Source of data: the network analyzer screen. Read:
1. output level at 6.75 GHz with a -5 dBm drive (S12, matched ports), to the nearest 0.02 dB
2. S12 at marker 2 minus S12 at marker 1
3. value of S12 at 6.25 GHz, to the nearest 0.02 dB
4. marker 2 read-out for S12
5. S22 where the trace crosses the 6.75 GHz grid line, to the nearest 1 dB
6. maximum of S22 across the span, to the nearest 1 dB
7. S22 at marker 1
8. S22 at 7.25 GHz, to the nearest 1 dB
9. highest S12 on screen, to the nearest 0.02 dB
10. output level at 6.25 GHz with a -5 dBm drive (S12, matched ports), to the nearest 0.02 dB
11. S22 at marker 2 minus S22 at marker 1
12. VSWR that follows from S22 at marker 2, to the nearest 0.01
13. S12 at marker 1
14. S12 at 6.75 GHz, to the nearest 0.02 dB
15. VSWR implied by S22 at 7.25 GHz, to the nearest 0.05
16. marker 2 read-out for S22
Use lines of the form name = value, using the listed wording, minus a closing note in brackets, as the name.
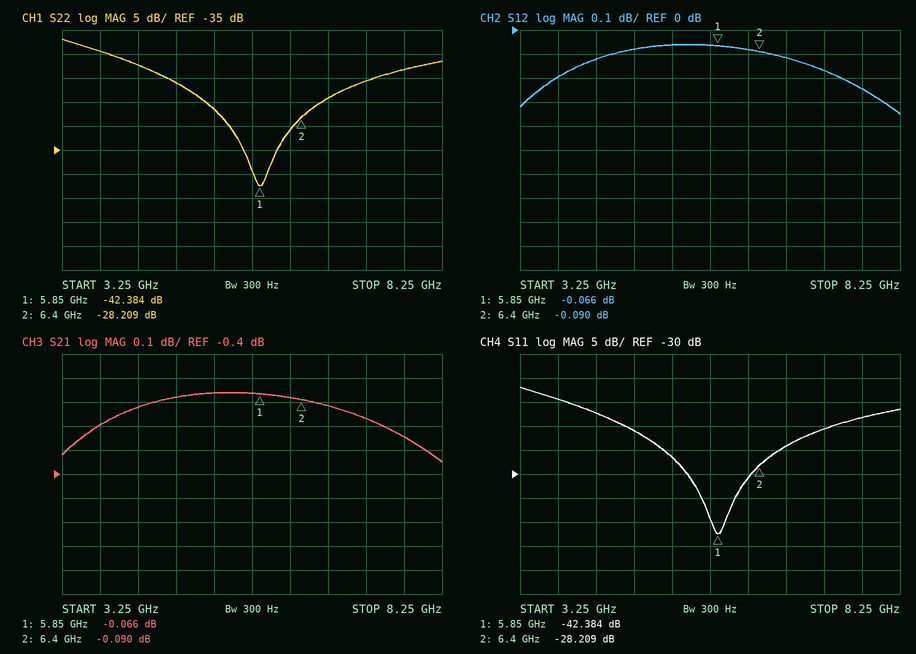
output level at 6.75 GHz with a -5 dBm drive (S12, matched ports), to the nearest 0.02 dB = -5.12 dBm
S12 at marker 2 minus S12 at marker 1 = -0.024 dB
value of S12 at 6.25 GHz, to the nearest 0.02 dB = -0.08 dB
marker 2 read-out for S12 = -0.090 dB
S22 where the trace crosses the 6.75 GHz grid line, to the nearest 1 dB = -24 dB
maximum of S22 across the span, to the nearest 1 dB = -12 dB
S22 at marker 1 = -42.384 dB
S22 at 7.25 GHz, to the nearest 1 dB = -21 dB
highest S12 on screen, to the nearest 0.02 dB = -0.06 dB
output level at 6.25 GHz with a -5 dBm drive (S12, matched ports), to the nearest 0.02 dB = -5.08 dBm
S22 at marker 2 minus S22 at marker 1 = 14.175 dB
VSWR that follows from S22 at marker 2, to the nearest 0.01 = 1.08
S12 at marker 1 = -0.066 dB
S12 at 6.75 GHz, to the nearest 0.02 dB = -0.12 dB
VSWR implied by S22 at 7.25 GHz, to the nearest 0.05 = 1.20
marker 2 read-out for S22 = -28.209 dB
